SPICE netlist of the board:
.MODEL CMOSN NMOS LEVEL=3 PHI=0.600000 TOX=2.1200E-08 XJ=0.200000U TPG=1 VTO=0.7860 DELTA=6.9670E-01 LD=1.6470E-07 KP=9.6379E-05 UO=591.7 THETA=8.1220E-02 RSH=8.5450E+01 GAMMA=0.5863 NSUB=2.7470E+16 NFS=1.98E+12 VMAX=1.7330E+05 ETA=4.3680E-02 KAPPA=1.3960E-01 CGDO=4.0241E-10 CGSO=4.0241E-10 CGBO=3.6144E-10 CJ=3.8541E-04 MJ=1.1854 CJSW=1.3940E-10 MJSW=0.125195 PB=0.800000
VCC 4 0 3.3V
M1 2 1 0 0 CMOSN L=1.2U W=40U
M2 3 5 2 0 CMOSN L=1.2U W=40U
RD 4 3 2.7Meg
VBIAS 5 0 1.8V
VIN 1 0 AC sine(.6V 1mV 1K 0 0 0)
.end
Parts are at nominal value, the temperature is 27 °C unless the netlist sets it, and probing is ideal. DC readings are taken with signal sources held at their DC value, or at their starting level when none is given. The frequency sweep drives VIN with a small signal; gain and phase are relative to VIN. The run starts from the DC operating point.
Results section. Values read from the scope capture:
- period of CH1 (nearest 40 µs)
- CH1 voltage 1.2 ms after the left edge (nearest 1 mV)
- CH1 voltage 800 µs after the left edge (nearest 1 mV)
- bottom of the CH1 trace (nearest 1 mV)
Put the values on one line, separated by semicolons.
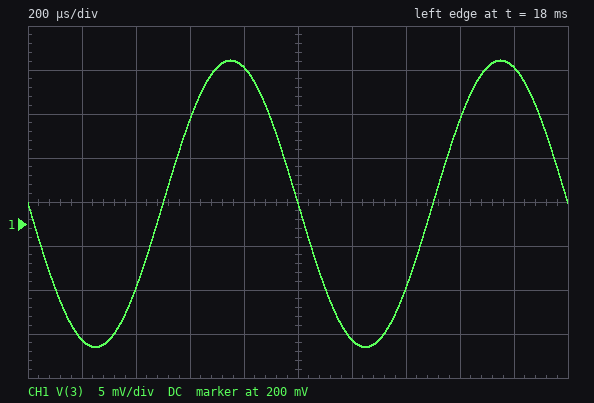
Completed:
1.00 ms; 187 mV; 218 mV; 186 mV
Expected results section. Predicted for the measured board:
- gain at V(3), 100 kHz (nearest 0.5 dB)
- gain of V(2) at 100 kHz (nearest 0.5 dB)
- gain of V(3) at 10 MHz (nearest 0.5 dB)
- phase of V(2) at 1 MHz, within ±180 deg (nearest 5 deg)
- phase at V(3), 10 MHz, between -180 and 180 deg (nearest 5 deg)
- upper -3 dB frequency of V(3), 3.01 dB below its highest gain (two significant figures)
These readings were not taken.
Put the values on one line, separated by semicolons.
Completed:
24.0 dB; 24.0 dB; 6.0 dB; 140 deg; 95 deg; 1.3 MHz
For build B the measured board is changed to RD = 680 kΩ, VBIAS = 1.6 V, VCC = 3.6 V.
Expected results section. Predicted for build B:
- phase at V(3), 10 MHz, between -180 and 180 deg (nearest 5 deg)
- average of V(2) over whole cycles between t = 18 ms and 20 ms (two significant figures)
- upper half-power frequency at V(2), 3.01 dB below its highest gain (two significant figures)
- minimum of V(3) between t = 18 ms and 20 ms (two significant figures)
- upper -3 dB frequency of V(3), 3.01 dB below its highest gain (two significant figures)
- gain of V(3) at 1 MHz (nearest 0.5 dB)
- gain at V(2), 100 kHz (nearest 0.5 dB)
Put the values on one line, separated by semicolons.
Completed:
135 deg; 840 mV; 27 MHz; 2.6 V; 13 MHz; 21.0 dB; 0.5 dB
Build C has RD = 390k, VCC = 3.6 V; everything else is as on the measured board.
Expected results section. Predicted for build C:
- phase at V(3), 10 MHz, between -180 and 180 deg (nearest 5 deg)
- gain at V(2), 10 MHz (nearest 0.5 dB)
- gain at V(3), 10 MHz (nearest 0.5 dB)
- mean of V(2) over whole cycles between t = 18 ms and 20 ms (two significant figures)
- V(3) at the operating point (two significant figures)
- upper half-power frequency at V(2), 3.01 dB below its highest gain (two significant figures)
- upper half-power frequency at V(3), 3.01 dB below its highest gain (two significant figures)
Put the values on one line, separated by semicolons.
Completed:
145 deg; -0.5 dB; 16.0 dB; 1.0 V; 3.0 V; 48 MHz; 22 MHz
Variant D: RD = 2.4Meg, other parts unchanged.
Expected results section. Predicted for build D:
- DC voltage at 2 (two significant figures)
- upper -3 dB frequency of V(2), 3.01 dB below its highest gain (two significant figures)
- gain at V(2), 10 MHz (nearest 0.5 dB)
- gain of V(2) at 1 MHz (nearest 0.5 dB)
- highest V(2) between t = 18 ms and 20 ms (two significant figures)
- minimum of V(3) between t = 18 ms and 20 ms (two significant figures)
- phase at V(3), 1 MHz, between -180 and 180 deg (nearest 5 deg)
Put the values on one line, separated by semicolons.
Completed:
360 mV; 1.4 MHz; 6.5 dB; 22.0 dB; 380 mV; 350 mV; 145 deg
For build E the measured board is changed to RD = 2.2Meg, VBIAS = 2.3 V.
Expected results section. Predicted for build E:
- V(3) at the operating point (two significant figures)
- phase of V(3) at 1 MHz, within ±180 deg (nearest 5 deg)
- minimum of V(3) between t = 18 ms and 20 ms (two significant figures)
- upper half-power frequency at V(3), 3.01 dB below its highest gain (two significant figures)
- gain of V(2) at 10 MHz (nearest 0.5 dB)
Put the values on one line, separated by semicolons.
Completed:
480 mV; 145 deg; 460 mV; 1.5 MHz; 7.0 dB
